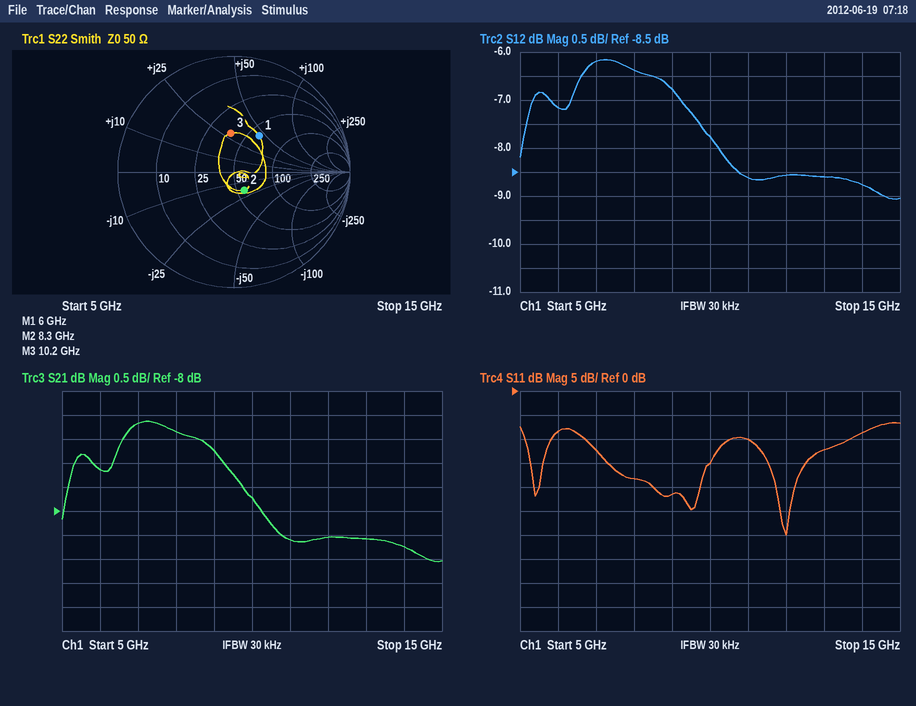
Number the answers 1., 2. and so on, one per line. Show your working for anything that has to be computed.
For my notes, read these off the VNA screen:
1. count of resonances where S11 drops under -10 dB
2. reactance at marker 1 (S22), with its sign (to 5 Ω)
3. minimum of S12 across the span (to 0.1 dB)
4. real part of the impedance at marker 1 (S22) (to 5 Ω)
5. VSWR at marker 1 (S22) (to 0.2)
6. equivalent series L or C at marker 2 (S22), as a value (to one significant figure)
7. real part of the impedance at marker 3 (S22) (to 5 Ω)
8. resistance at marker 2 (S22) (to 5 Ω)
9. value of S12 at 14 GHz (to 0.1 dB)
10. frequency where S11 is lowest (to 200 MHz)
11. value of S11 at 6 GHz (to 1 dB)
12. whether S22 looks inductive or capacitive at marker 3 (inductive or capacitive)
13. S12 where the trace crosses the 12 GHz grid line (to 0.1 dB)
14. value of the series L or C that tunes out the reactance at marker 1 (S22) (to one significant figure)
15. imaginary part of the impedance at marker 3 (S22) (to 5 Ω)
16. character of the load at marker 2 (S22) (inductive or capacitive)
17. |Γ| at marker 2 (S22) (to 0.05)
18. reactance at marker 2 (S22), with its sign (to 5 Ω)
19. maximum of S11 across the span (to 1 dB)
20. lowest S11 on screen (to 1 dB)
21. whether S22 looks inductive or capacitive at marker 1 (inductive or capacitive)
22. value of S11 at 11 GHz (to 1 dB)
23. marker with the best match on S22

1. 3
2. +45 Ω
3. -9.1 dB
4. 60 Ω
5. 2.2
6. C = 1/(2π × 8.3 GHz × 20 Ω) ≈ 1 pF
7. 40 Ω
8. 55 Ω
9. -8.8 dB
10. 12.0 GHz
11. -8 dB
12. inductive
13. -8.6 dB
14. C = 1/(2π × 6 GHz × 45 Ω) ≈ 589 fF, so 600 fF to one significant figure
15. +30 Ω
16. capacitive
17. 0.20
18. -20 Ω
19. -7 dB
20. -30 dB
21. inductive
22. -10 dB
23. marker 2
